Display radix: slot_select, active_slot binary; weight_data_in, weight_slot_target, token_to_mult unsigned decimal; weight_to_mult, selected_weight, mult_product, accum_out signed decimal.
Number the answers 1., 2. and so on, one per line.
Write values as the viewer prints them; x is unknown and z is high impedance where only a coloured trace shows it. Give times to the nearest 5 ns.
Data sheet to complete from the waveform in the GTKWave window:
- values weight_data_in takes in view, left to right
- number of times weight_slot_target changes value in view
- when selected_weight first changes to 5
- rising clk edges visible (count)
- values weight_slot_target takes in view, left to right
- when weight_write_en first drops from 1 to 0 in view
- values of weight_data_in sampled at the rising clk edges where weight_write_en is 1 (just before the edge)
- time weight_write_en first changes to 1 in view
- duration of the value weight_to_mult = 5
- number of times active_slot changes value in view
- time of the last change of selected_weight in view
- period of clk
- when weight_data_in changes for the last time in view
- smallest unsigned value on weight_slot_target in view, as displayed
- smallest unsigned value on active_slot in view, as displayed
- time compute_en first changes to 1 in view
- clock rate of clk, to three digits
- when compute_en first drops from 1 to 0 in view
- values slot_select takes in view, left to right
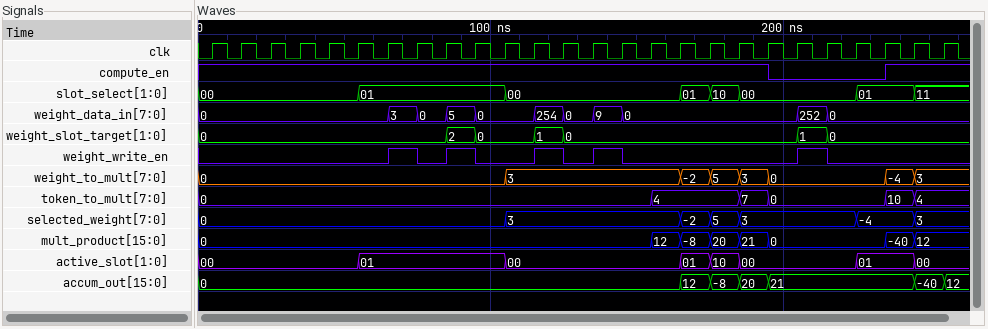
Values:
1. 0, 3, 0, 5, 0, 254, 0, 9, 0, 252, 0
2. 6
3. 175 ns
4. 26
5. 0, 2, 0, 1, 0, 1, 0
6. 75 ns
7. 3, 5, 254, 9, 252
8. 65 ns
9. 10 ns
10. 7
11. 245 ns
12. 10 ns
13. 215 ns
14. 0
15. 00
16. 235 ns
17. 100 MHz
18. 195 ns
19. 00, 01, 00, 01, 10, 00, 01, 11
